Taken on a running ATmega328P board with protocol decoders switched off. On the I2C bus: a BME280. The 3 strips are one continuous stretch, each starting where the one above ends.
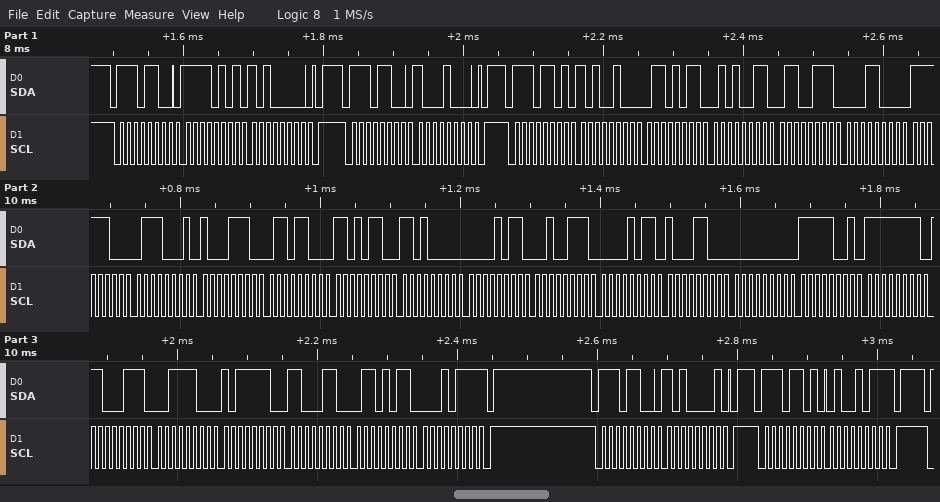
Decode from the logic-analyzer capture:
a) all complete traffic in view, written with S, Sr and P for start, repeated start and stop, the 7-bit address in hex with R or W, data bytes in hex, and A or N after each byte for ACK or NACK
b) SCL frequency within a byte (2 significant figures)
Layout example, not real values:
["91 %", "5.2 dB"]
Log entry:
["S 76W A F5 A A0 A P S 76W A 88 A P S 76R A A4 A 6B A 53 A 67 A 18 A FC A 71 A 8E A 6C A D6 A D0 A 0B A 27 A 0B A 8C A 00 A F9 A FF A C7 A 3C A BE A C6 A 6B A 17 N P S 76W A A1 A P S 76R A 4B N P", "100 kHz"]
